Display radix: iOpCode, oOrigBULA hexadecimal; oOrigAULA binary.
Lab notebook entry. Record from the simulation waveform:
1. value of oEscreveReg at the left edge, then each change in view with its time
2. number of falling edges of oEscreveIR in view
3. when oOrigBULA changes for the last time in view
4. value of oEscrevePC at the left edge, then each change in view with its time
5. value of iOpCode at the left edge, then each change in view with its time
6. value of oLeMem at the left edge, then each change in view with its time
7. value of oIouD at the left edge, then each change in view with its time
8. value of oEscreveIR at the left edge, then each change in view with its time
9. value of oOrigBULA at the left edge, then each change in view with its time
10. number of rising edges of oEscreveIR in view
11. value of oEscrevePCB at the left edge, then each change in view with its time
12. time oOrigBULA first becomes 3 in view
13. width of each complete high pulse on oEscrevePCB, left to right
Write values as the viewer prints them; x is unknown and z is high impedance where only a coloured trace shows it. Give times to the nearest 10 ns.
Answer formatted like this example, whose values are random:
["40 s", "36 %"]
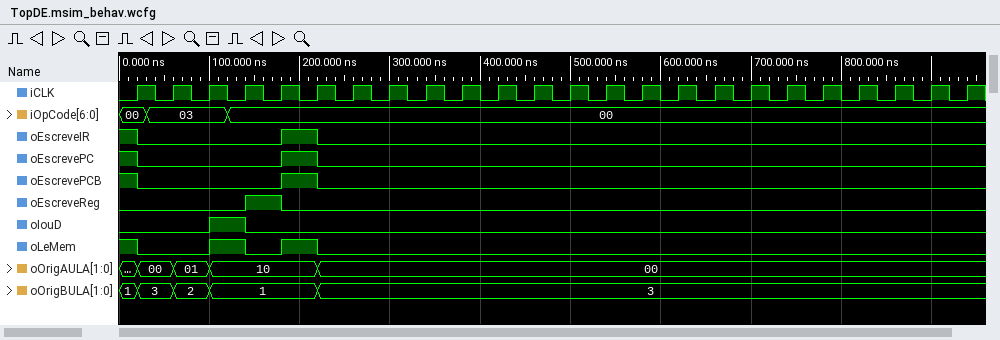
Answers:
["0, 1 at 140 ns, 0 at 180 ns", "2", "220 ns", "1, 0 at 20 ns, 1 at 180 ns, 0 at 220 ns", "00, 03 at 30 ns, 00 at 120 ns", "1, 0 at 20 ns, 1 at 100 ns, 0 at 140 ns, 1 at 180 ns, 0 at 220 ns", "0, 1 at 100 ns, 0 at 140 ns", "1, 0 at 20 ns, 1 at 180 ns, 0 at 220 ns", "1, 3 at 20 ns, 2 at 60 ns, 1 at 100 ns, 3 at 220 ns", "1", "1, 0 at 20 ns, 1 at 180 ns, 0 at 220 ns", "20 ns", "40 ns"]
